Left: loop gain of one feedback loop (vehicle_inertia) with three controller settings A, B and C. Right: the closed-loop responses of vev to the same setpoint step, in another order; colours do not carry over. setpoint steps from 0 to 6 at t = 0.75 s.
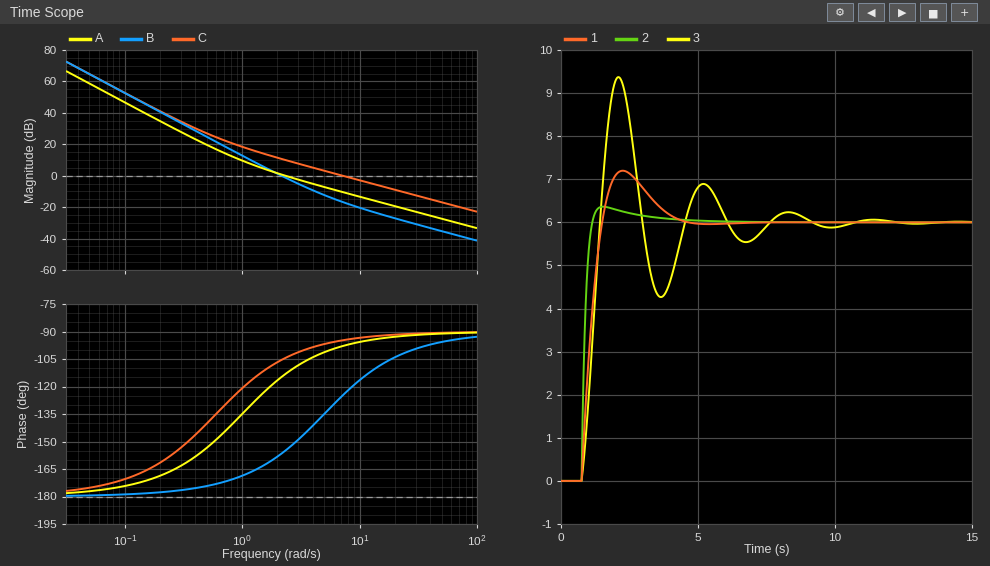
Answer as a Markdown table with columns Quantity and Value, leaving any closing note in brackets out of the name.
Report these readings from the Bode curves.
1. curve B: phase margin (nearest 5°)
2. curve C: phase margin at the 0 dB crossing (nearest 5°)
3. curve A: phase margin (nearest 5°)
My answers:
| Quantity | Value |
|---|---|
| curve B: phase margin | 25° |
| curve C: phase margin at the 0 dB crossing | 85° |
| curve A: phase margin | 65° |
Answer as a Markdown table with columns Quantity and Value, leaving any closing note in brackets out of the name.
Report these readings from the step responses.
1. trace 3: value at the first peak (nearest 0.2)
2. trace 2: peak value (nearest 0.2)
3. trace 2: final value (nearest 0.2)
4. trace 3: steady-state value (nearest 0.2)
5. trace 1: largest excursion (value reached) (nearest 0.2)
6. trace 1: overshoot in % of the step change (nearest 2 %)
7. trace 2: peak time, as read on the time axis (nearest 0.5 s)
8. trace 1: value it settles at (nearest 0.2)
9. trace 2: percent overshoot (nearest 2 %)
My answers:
| Quantity | Value |
|---|---|
| trace 3: value at the first peak | 9.4 |
| trace 2: peak value | 6.4 |
| trace 2: final value | 6.0 |
| trace 3: steady-state value | 6.0 |
| trace 1: largest excursion (value reached) | 7.2 |
| trace 1: overshoot in % of the step change | 20 % |
| trace 2: peak time, as read on the time axis | 1.5 s |
| trace 1: value it settles at | 6.0 |
| trace 2: percent overshoot | 6 % |
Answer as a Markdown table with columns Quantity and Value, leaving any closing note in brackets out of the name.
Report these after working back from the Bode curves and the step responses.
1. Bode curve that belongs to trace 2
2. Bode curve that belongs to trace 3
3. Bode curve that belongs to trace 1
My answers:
| Quantity | Value |
|---|---|
| Bode curve that belongs to trace 2 | C |
| Bode curve that belongs to trace 3 | B |
| Bode curve that belongs to trace 1 | A |
